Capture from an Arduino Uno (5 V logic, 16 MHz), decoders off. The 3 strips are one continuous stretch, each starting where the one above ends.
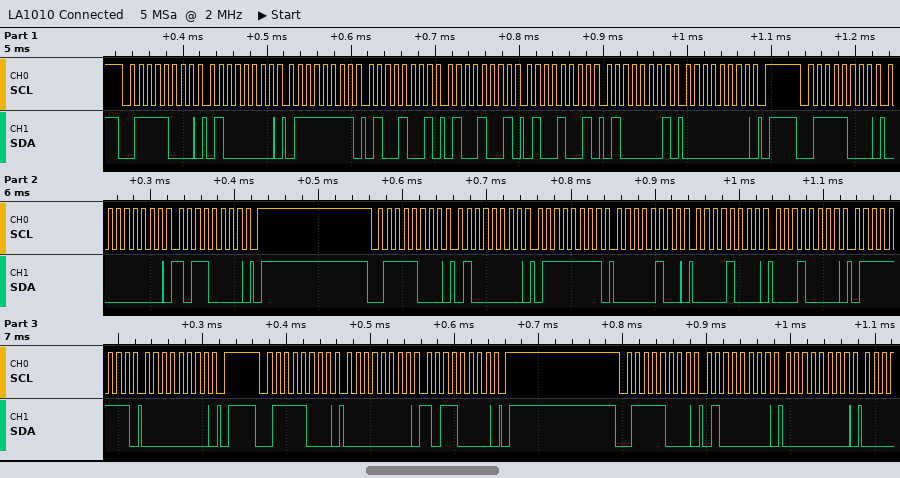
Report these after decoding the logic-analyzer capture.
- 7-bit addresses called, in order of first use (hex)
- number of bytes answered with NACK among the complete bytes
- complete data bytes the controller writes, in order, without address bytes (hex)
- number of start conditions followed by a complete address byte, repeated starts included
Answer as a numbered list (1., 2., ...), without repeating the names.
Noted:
1. 0x3C
2. 0
3. 40 7F 49 49 49 41 00 00 B0 40 7F 04 08 10 7F 00 00 B0 40 00
4. 5
